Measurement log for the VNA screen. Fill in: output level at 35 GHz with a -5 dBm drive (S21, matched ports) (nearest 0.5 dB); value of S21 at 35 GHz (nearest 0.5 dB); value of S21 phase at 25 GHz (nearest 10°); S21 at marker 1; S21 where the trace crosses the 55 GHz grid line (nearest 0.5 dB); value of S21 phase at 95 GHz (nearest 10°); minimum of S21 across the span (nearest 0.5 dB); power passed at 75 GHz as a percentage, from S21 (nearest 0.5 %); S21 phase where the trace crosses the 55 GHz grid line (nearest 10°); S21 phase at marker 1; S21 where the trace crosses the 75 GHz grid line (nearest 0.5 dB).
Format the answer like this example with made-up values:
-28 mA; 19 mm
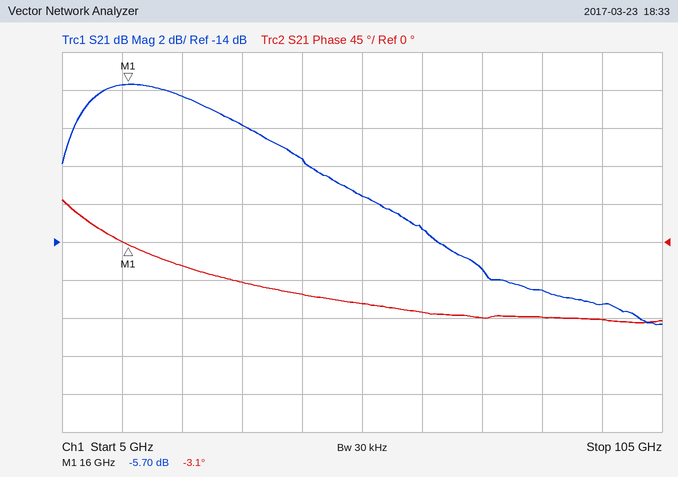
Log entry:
-13.0 dBm; -8.0 dB; -30°; -5.70 dB; -11.5 dB; -90°; -18.5 dB; 3.0 %; -70°; -3.1°; -15.5 dB
